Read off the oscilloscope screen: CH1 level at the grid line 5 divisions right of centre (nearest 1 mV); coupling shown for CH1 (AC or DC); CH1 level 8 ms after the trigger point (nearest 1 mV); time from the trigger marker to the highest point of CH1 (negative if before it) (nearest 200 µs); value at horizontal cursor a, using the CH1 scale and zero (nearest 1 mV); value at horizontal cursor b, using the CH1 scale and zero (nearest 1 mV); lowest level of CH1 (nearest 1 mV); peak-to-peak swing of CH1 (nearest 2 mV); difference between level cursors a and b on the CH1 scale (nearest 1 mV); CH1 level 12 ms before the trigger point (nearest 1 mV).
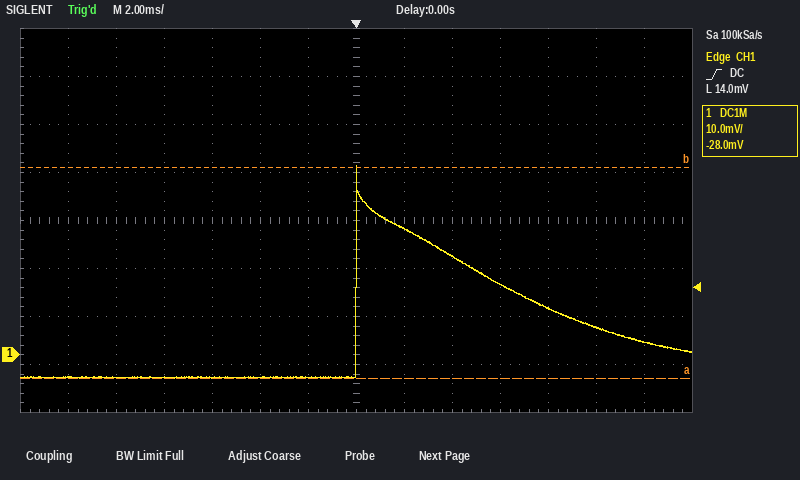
6 mV
DC
10 mV
0.0 ms
-5 mV
39 mV
-5 mV
44 mV
44 mV
-5 mV
